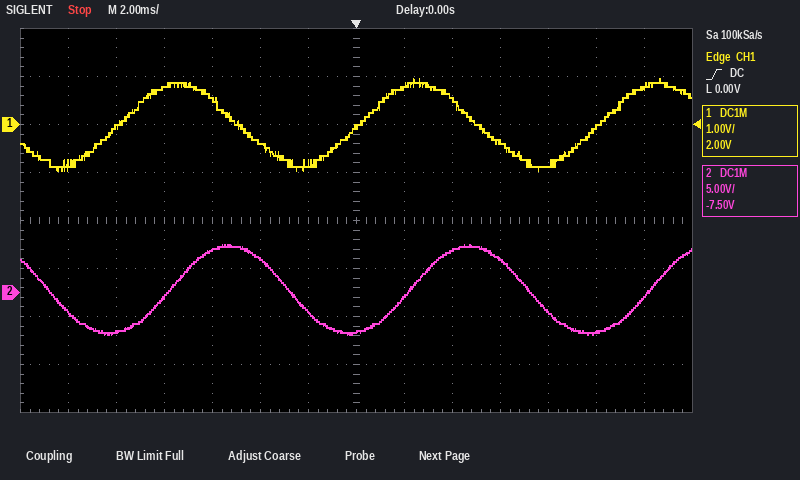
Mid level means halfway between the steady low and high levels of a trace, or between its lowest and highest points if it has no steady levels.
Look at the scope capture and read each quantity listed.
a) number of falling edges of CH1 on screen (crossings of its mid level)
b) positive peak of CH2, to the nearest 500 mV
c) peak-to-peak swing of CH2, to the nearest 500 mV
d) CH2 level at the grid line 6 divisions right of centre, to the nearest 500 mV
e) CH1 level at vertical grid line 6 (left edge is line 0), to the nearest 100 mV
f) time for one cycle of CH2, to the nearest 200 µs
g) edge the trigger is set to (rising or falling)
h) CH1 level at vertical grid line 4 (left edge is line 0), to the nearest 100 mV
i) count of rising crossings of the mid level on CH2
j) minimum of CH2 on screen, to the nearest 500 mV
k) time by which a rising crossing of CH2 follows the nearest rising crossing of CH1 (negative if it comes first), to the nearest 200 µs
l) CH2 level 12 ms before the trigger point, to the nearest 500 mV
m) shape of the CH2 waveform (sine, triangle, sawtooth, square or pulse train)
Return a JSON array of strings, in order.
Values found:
["2", "5.0 V", "9.5 V", "-500 mV", "-800 mV", "10.0 ms", "rising", "500 mV", "3", "-4.5 V", "+2.2 ms", "-2.0 V", "sine"]
